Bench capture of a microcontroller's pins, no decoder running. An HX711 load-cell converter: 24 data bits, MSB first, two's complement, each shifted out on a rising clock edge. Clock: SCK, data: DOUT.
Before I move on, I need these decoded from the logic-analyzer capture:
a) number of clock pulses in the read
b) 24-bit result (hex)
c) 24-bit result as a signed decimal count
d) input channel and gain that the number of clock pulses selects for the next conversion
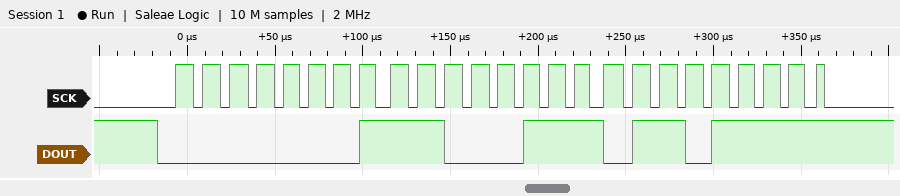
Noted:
25
0x01C76F
116591
channel A, gain 128
